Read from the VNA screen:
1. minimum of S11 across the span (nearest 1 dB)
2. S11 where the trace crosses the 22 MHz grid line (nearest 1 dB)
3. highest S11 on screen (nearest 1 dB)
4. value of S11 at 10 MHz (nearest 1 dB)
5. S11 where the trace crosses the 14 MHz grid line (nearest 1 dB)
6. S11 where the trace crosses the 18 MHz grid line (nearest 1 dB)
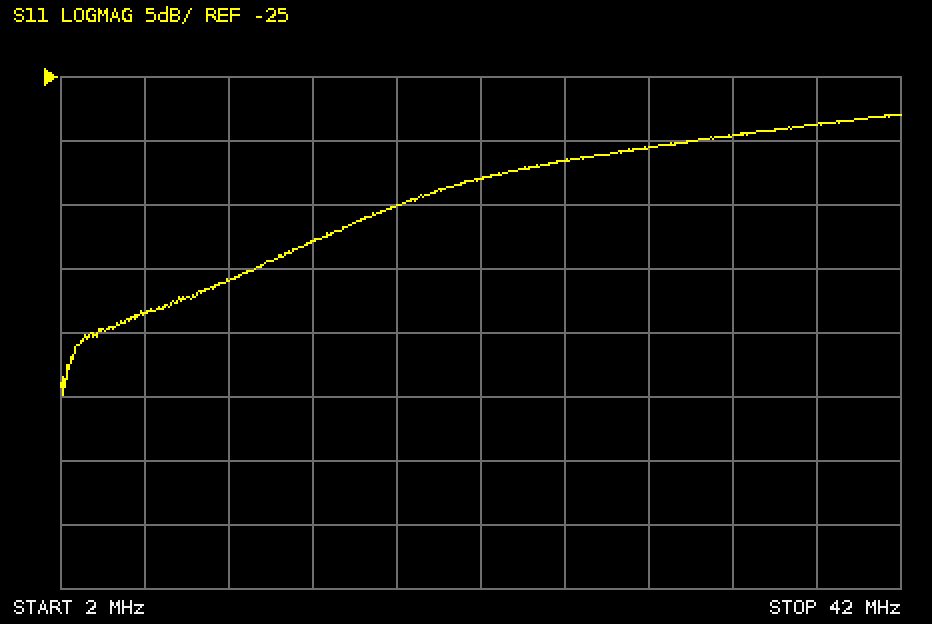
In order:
-50 dB
-33 dB
-28 dB
-41 dB
-38 dB
-35 dB
